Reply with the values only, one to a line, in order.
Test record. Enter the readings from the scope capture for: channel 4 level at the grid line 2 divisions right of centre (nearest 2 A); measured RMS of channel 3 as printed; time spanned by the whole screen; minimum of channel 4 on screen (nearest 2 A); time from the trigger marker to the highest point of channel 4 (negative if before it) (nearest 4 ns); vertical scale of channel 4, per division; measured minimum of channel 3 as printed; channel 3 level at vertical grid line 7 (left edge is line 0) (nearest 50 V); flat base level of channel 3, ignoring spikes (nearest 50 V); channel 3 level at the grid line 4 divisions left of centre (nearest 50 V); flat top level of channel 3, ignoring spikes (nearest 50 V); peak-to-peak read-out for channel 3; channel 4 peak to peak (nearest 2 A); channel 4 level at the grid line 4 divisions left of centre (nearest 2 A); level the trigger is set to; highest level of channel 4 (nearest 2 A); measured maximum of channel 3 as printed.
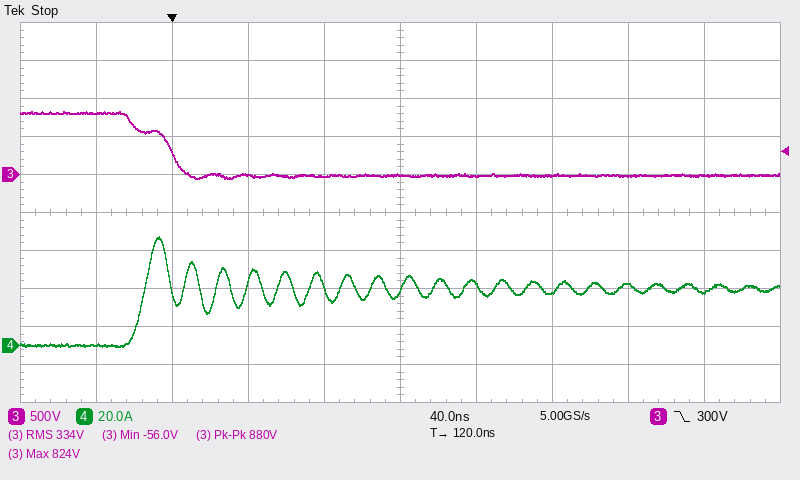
28 A
334 V
400 ns
0 A
-8 ns
20 A
-56.0 V
0 V
0 V
800 V
800 V
880 V
58 A
0 A
300 V
58 A
824 V
